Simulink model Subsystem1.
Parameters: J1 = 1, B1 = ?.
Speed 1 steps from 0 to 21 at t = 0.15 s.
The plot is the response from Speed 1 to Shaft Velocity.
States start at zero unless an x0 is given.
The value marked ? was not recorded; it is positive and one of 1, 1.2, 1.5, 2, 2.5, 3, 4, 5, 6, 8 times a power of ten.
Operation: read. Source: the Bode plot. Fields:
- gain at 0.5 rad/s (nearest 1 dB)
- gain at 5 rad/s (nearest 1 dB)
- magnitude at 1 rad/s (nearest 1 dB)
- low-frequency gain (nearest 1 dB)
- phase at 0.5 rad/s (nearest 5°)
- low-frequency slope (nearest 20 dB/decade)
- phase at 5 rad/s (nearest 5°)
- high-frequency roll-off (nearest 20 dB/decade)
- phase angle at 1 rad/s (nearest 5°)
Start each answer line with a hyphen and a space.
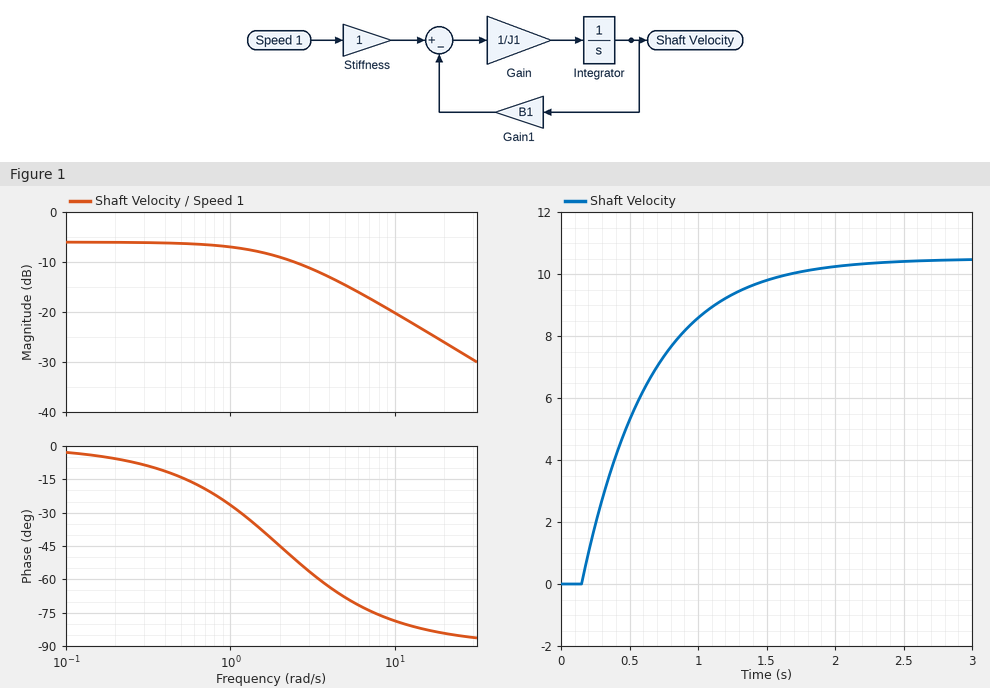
- -6 dB
- -15 dB
- -7 dB
- -6 dB
- -15°
- 0 dB/decade
- -70°
- -20 dB/decade
- -25°
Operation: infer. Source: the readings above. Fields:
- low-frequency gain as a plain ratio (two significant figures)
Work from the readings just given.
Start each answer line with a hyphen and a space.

- 0.50
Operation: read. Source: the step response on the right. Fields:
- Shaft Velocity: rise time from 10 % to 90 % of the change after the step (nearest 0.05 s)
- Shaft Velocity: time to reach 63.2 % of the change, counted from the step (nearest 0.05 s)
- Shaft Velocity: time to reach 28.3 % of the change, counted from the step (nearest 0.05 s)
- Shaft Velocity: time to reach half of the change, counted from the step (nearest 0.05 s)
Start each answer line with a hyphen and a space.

- 1.10 s
- 0.50 s
- 0.15 s
- 0.35 s
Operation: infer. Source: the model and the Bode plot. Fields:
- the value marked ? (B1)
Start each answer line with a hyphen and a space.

- 2
